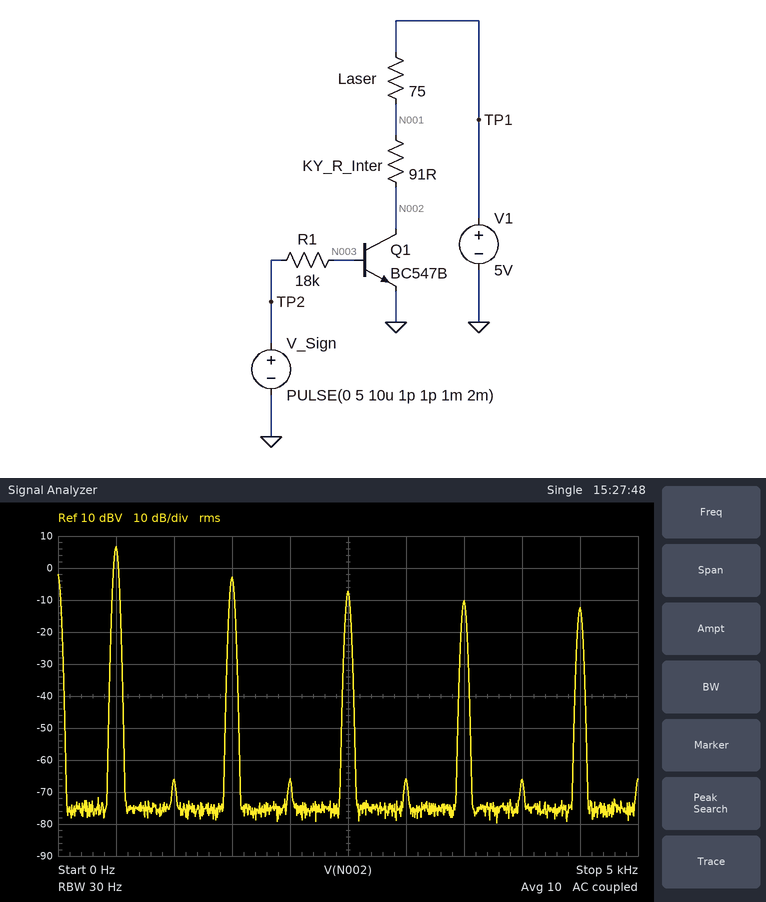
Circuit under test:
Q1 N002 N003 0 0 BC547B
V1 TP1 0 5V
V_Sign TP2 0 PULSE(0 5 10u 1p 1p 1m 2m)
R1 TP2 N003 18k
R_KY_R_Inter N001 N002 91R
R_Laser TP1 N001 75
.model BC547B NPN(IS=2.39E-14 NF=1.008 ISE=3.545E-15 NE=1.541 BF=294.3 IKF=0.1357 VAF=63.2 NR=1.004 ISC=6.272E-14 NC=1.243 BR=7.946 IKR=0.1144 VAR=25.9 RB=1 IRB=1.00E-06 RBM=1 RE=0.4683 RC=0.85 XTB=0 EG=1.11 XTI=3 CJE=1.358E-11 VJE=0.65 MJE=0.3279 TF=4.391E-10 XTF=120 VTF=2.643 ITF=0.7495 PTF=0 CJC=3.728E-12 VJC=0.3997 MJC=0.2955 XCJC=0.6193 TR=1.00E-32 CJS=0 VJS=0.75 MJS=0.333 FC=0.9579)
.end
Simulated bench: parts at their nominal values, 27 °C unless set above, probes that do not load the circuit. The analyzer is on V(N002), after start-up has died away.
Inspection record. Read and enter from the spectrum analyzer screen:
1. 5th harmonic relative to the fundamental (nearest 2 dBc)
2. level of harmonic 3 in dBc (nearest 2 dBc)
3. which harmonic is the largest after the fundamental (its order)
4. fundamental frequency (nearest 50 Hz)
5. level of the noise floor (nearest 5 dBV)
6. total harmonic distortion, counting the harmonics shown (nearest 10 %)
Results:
-14 dBc
-10 dBc
3
500 Hz
-75 dBV
40 %
